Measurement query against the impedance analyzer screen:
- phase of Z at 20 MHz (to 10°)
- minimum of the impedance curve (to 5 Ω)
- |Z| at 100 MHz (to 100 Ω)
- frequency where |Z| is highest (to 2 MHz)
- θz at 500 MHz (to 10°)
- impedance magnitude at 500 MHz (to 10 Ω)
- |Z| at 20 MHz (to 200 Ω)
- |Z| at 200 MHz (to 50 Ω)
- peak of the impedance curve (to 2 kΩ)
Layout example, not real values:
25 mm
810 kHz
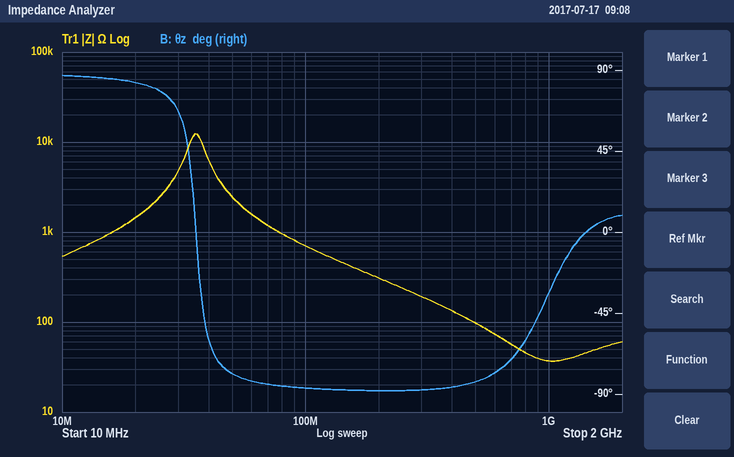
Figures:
80°
35 Ω
700 Ω
36 MHz
-80°
100 Ω
1.4 kΩ
300 Ω
12 kΩ
